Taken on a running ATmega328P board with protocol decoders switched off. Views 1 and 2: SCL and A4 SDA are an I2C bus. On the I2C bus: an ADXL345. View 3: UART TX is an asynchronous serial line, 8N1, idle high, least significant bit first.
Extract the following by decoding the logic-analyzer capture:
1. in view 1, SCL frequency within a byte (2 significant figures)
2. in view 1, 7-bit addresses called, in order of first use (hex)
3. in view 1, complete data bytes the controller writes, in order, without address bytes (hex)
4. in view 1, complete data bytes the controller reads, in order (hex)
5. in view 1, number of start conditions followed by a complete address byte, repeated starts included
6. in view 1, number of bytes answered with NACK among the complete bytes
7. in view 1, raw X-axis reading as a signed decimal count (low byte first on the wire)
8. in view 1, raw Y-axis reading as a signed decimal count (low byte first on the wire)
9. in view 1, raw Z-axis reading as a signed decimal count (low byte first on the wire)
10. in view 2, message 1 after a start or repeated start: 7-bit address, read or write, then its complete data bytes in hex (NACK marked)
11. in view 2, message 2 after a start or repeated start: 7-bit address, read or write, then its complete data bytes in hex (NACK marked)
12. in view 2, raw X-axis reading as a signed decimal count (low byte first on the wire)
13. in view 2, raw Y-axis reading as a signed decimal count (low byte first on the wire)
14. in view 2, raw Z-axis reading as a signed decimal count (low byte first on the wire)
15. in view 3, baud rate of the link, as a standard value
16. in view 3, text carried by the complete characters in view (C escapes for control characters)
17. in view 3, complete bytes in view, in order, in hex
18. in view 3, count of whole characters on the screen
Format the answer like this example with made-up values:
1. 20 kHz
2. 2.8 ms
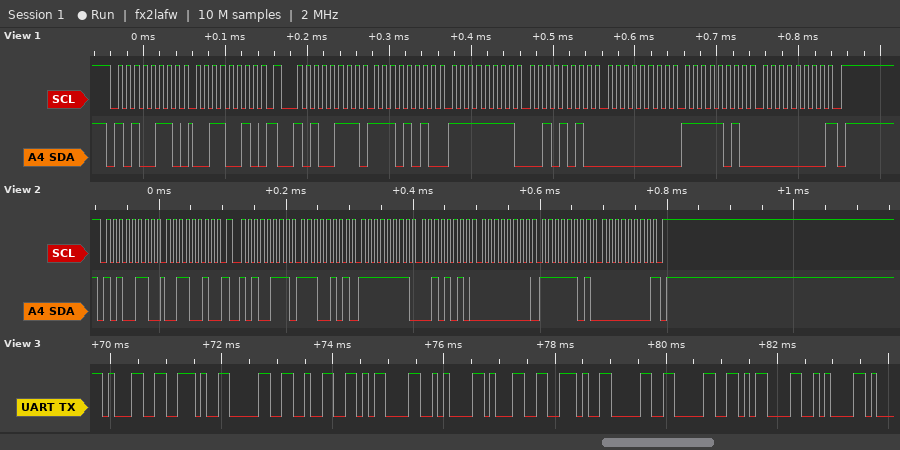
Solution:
1. 100 kHz
2. 0x53
3. 32
4. EA FF 2A 00 FA 00
5. 2
6. 1
7. -22
8. 42
9. 250
10. 0x53 write: 32
11. 0x53 read: E5 FF 2A 00 FD 00 NACK
12. -27
13. 42
14. 253
15. 9600 baud
16. "1.02\r\n1.00\r\n"
17. 31 2E 30 32 0D 0A 31 2E 30 30 0D 0A
18. 12
